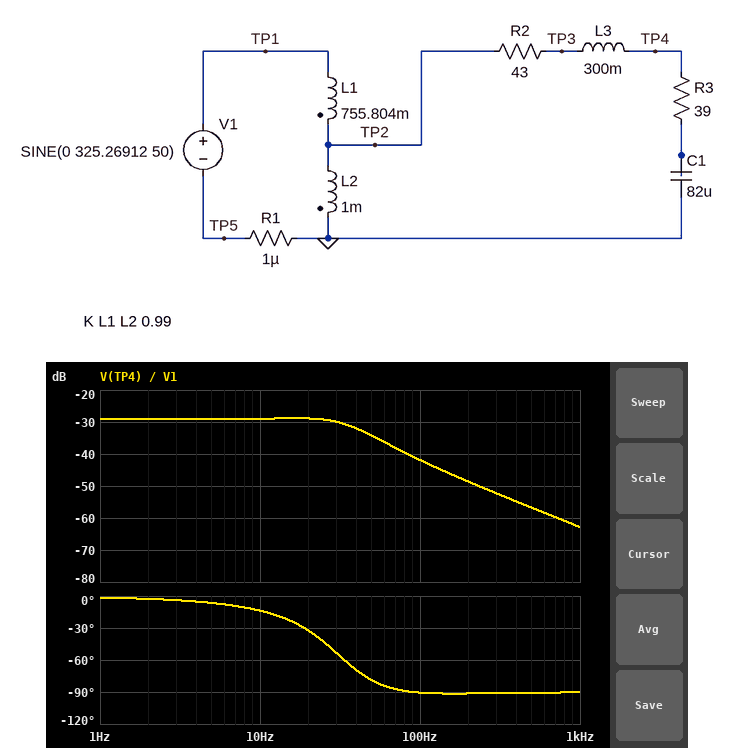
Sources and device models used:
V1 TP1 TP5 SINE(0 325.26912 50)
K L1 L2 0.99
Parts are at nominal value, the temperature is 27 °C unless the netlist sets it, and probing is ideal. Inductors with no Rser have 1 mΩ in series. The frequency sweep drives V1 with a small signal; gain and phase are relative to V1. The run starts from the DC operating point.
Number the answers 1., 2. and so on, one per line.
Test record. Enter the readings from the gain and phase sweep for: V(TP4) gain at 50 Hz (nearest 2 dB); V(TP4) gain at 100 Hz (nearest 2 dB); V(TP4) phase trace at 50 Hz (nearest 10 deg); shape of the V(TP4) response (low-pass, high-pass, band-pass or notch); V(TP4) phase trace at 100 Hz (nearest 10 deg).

1. -34 dB
2. -42 dB
3. -80 deg
4. low-pass
5. -90 deg
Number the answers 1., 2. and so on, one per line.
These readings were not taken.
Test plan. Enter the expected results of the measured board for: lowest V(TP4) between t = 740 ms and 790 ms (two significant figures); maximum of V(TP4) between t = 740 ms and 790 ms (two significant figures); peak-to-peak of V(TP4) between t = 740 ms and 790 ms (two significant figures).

1. -6.3 V
2. 6.3 V
3. 13 V
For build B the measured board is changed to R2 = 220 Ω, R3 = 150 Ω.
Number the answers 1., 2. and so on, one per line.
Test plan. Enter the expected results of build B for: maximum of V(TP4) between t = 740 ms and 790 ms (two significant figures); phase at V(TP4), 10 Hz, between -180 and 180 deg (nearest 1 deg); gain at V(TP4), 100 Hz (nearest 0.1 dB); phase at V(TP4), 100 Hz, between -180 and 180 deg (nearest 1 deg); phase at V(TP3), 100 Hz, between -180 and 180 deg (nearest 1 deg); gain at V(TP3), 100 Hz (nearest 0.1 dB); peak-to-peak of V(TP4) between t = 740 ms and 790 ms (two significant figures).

1. 4.7 V
2. -27 deg
3. -37.8 dB
4. -32 deg
5. 24 deg
6. -34.3 dB
7. 9.4 V
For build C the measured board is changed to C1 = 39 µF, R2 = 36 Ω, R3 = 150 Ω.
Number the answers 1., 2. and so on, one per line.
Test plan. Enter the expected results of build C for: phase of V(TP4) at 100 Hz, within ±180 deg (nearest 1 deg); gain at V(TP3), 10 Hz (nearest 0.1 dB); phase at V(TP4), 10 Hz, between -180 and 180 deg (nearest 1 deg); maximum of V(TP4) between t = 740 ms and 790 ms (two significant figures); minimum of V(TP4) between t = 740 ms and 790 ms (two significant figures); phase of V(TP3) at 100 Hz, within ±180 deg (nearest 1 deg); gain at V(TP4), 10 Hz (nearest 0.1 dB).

1. -54 deg
2. -29.5 dB
3. -5 deg
4. 10 V
5. -10 V
6. 6 deg
7. -29.1 dB
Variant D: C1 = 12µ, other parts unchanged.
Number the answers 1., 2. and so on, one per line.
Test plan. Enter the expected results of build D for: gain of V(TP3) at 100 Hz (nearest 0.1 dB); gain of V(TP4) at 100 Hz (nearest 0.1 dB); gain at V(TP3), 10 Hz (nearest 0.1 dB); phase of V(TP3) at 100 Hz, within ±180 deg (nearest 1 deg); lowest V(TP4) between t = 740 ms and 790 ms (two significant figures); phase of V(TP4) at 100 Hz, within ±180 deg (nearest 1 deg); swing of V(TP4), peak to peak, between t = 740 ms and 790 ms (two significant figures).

1. -32.4 dB
2. -26.3 dB
3. -29.2 dB
4. 21 deg
5. -16 V
6. -108 deg
7. 32 V
